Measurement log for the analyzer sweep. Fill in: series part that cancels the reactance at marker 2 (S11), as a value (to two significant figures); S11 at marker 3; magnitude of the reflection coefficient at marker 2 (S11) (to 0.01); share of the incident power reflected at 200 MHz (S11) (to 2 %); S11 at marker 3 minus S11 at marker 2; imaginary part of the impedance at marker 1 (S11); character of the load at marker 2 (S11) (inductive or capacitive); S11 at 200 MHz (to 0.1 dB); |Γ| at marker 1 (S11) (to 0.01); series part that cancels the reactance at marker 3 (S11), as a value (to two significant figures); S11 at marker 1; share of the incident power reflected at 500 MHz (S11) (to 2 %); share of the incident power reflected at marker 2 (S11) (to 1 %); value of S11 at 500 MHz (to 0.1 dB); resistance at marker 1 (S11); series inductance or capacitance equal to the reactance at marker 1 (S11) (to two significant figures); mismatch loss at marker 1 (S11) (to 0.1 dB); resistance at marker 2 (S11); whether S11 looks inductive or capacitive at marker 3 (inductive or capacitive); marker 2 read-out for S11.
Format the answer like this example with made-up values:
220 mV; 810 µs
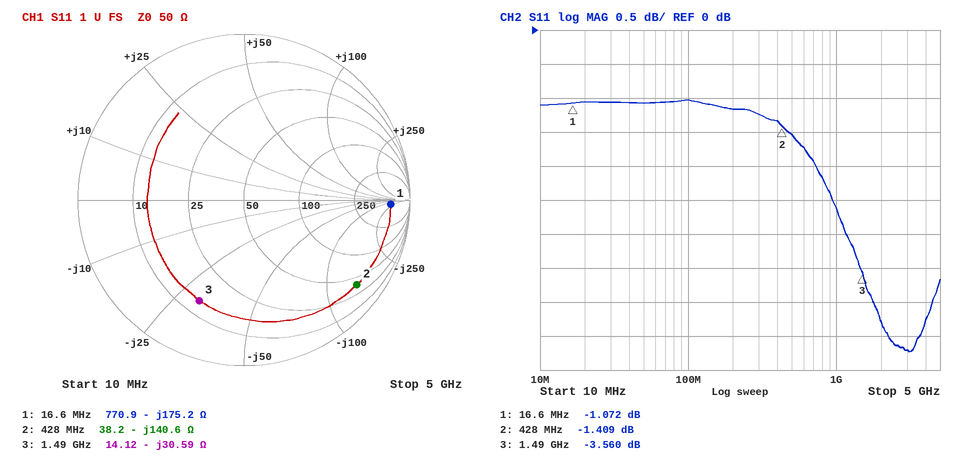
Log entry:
52 nH; -3.560 dB; 0.85; 76 %; -2.151 dB; -175.2 Ω; capacitive; -1.2 dB; 0.88; 3.3 nH; -1.072 dB; 70 %; 72 %; -1.5 dB; 770.9 Ω; 55 pF; 6.6 dB; 38.2 Ω; capacitive; -1.409 dB
